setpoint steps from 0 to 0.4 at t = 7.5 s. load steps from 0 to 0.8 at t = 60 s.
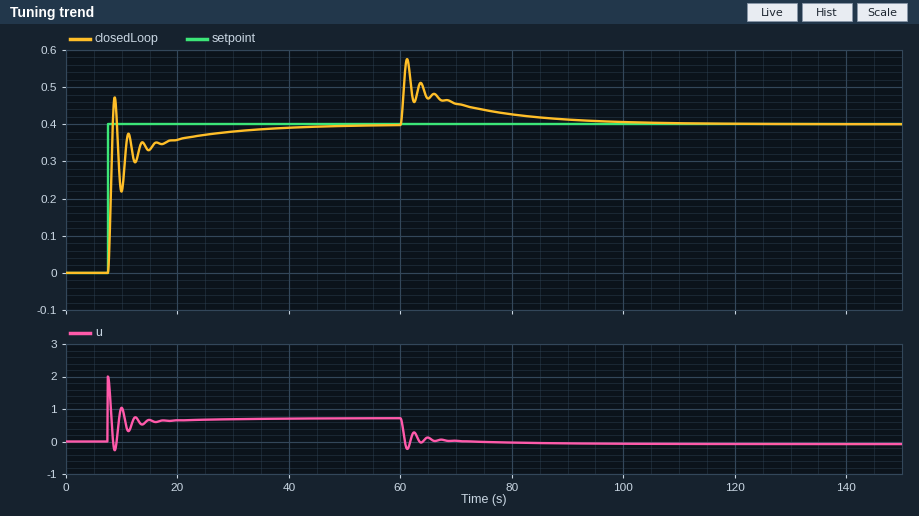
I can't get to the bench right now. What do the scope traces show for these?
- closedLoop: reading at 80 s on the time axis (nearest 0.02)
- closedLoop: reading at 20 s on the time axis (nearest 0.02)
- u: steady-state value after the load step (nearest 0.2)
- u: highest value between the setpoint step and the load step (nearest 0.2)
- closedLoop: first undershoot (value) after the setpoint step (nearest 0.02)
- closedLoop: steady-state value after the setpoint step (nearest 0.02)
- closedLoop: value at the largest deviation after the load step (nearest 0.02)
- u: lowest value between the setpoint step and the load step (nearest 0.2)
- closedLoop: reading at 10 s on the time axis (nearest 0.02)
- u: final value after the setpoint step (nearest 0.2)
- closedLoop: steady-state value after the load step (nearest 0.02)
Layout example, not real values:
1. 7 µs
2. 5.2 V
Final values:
1. 0.42
2. 0.36
3. 0.0
4. 2.0
5. 0.22
6. 0.40
7. 0.58
8. -0.2
9. 0.22
10. 0.8
11. 0.40
